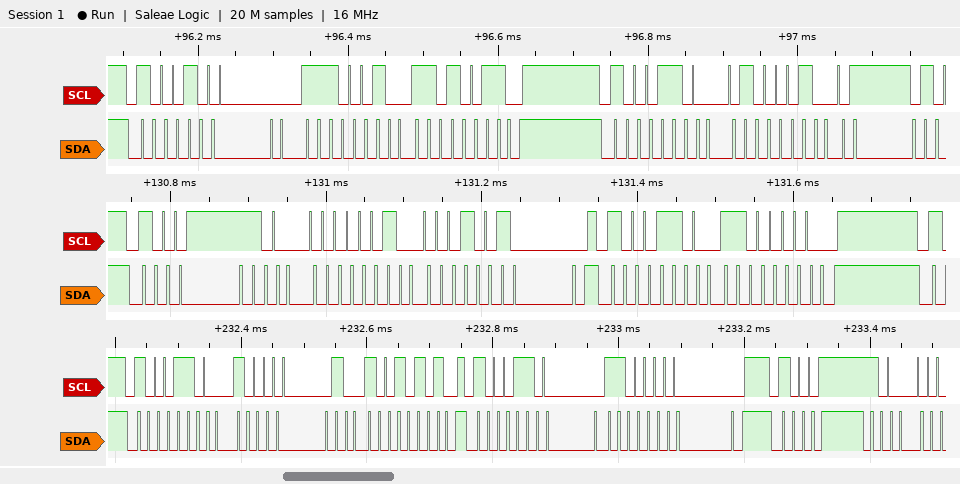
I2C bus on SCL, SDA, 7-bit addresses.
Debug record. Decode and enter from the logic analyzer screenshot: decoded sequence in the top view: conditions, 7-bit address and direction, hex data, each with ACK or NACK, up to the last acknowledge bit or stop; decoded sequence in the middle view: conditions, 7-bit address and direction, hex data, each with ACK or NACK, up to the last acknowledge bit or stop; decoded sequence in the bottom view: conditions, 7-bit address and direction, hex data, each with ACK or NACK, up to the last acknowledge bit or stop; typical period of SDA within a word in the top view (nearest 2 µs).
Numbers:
start, address 44 write ACK, E2 ACK, D3 ACK, stop, start, address 46 write ACK, 42 ACK
start, address 46 write ACK, 02 ACK, 12 ACK, stop, start, address 46 write ACK, C0 ACK, stop
start, address 46 write ACK, 82 ACK, 95 ACK, stop, start, address 46 write ACK, C0 ACK, stop, start, address 46 write ACK
16 µs
